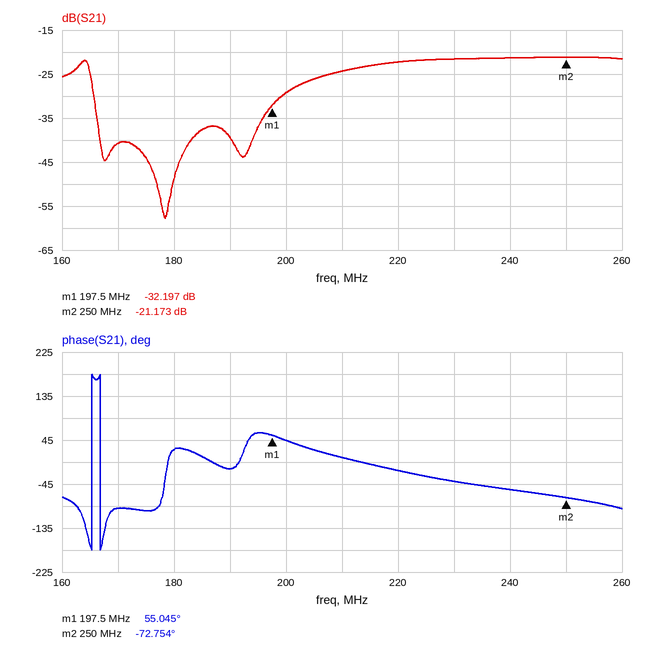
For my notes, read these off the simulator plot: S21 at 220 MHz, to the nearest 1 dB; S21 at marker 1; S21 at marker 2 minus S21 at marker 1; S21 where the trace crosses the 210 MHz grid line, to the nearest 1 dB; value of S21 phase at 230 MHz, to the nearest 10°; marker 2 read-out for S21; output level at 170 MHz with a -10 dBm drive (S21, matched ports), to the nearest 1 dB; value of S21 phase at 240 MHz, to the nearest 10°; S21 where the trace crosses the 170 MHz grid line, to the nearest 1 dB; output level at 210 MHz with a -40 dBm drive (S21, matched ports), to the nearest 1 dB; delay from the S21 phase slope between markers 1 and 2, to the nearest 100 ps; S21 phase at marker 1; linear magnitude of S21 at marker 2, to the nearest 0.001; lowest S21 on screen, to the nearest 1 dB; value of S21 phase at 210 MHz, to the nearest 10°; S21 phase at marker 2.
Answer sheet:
-22 dB
-32.197 dB
11.024 dB
-24 dB
-40°
-21.173 dB
-51 dBm
-60°
-41 dB
-64 dBm
6.8 ns
55.045°
0.087
-58 dB
10°
-72.754°
